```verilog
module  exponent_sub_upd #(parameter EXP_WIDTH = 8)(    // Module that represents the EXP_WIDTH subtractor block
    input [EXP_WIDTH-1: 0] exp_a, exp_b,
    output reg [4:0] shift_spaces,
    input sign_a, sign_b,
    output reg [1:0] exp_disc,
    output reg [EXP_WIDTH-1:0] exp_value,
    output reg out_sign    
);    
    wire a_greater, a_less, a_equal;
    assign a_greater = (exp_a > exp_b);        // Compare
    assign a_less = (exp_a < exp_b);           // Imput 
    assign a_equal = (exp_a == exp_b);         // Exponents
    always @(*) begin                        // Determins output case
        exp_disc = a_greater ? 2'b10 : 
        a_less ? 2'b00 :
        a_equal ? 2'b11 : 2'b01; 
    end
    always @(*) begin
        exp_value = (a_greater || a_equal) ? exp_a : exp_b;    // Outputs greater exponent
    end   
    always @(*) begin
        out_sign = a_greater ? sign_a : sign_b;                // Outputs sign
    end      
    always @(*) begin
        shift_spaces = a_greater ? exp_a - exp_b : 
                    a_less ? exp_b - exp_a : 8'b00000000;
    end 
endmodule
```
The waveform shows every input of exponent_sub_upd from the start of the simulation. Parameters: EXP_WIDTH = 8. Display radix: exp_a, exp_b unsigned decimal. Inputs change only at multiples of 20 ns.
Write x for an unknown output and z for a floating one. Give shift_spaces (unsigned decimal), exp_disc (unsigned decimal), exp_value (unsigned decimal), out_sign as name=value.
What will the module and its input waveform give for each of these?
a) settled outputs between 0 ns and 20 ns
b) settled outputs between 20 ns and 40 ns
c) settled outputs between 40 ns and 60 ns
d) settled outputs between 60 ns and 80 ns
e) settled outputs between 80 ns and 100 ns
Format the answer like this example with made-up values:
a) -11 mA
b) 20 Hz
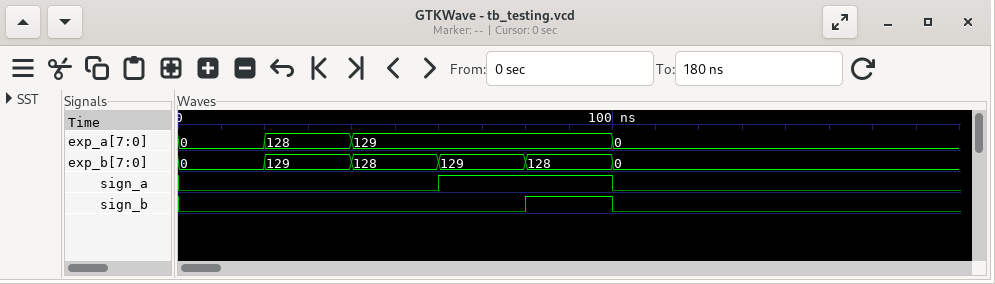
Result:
a) shift_spaces=0, exp_disc=3, exp_value=0, out_sign=0
b) shift_spaces=1, exp_disc=0, exp_value=129, out_sign=0
c) shift_spaces=1, exp_disc=2, exp_value=129, out_sign=0
d) shift_spaces=0, exp_disc=3, exp_value=129, out_sign=0
e) shift_spaces=1, exp_disc=2, exp_value=129, out_sign=1
